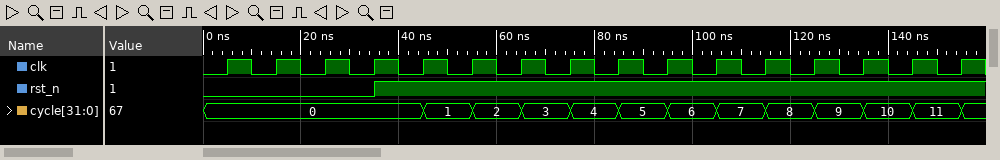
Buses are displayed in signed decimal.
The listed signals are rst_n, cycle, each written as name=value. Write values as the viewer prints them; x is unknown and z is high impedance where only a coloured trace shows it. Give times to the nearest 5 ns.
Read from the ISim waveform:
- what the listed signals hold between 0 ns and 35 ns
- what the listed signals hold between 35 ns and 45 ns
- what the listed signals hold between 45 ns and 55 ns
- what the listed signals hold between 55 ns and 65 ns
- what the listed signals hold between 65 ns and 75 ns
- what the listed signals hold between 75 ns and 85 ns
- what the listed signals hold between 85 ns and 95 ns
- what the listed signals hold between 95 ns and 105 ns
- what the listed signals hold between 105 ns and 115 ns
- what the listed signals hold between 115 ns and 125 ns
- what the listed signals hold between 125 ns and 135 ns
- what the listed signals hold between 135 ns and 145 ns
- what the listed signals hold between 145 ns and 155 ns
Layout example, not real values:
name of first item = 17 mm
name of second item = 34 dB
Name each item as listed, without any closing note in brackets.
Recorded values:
what the listed signals hold between 0 ns and 35 ns = rst_n=0, cycle=0
what the listed signals hold between 35 ns and 45 ns = rst_n=1, cycle=0
what the listed signals hold between 45 ns and 55 ns = rst_n=1, cycle=1
what the listed signals hold between 55 ns and 65 ns = rst_n=1, cycle=2
what the listed signals hold between 65 ns and 75 ns = rst_n=1, cycle=3
what the listed signals hold between 75 ns and 85 ns = rst_n=1, cycle=4
what the listed signals hold between 85 ns and 95 ns = rst_n=1, cycle=5
what the listed signals hold between 95 ns and 105 ns = rst_n=1, cycle=6
what the listed signals hold between 105 ns and 115 ns = rst_n=1, cycle=7
what the listed signals hold between 115 ns and 125 ns = rst_n=1, cycle=8
what the listed signals hold between 125 ns and 135 ns = rst_n=1, cycle=9
what the listed signals hold between 135 ns and 145 ns = rst_n=1, cycle=10
what the listed signals hold between 145 ns and 155 ns = rst_n=1, cycle=11
